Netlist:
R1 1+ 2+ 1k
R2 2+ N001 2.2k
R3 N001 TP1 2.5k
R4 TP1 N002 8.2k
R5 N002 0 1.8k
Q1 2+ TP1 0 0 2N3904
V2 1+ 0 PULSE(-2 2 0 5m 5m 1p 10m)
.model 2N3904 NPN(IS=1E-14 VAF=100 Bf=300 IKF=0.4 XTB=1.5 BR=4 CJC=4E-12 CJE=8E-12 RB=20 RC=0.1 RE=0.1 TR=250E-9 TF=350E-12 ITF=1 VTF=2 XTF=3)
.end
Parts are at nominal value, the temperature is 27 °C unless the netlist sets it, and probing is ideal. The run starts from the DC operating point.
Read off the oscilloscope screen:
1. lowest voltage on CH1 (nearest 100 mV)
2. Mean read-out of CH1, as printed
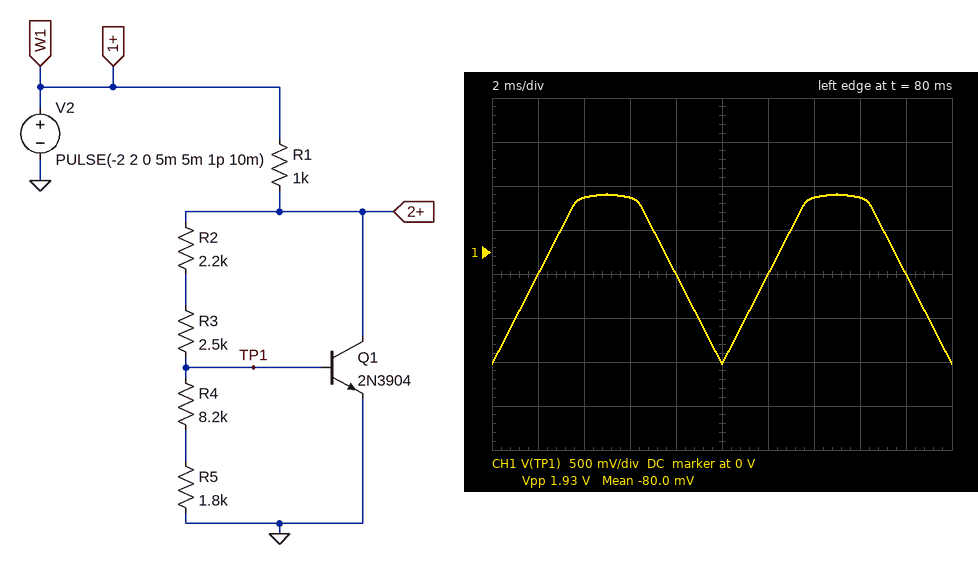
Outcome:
-1.3 V
-80.0 mV
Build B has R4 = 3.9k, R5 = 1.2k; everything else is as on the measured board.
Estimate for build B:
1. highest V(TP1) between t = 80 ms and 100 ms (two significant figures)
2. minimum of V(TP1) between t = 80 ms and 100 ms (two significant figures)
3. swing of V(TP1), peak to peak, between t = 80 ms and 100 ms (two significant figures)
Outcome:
640 mV
-960 mV
1.6 V
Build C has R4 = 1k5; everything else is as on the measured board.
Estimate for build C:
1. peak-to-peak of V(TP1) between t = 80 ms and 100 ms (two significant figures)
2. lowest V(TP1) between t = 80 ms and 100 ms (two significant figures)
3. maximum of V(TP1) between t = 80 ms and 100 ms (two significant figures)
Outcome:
1.4 V
-760 mV
620 mV
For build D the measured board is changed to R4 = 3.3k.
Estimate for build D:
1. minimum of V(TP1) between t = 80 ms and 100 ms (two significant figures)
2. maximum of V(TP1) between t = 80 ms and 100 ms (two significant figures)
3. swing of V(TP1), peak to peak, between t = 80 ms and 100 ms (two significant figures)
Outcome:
-960 mV
640 mV
1.6 V
